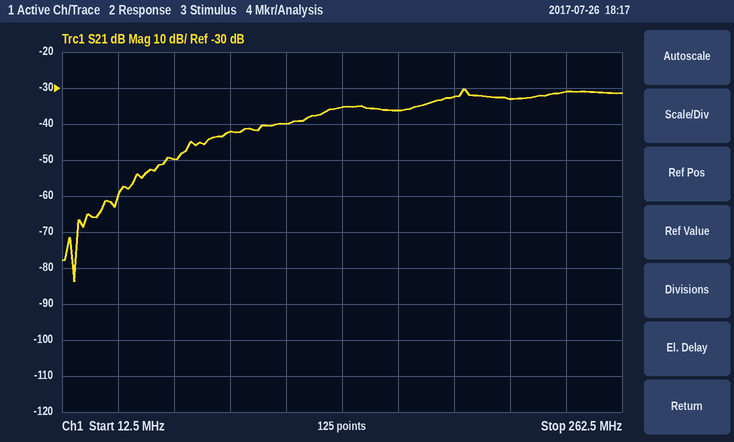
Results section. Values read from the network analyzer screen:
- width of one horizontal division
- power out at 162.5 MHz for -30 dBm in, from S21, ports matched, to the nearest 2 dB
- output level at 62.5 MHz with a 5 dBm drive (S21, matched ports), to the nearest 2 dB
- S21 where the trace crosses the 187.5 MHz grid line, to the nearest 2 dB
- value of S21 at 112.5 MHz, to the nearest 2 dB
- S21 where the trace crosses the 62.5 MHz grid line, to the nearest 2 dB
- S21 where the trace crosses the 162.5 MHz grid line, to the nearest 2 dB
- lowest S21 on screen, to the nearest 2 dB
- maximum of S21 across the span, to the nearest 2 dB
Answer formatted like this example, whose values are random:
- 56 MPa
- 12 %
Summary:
- 25 MHz
- -66 dBm
- -44 dBm
- -32 dB
- -40 dB
- -50 dB
- -36 dB
- -84 dB
- -30 dB
